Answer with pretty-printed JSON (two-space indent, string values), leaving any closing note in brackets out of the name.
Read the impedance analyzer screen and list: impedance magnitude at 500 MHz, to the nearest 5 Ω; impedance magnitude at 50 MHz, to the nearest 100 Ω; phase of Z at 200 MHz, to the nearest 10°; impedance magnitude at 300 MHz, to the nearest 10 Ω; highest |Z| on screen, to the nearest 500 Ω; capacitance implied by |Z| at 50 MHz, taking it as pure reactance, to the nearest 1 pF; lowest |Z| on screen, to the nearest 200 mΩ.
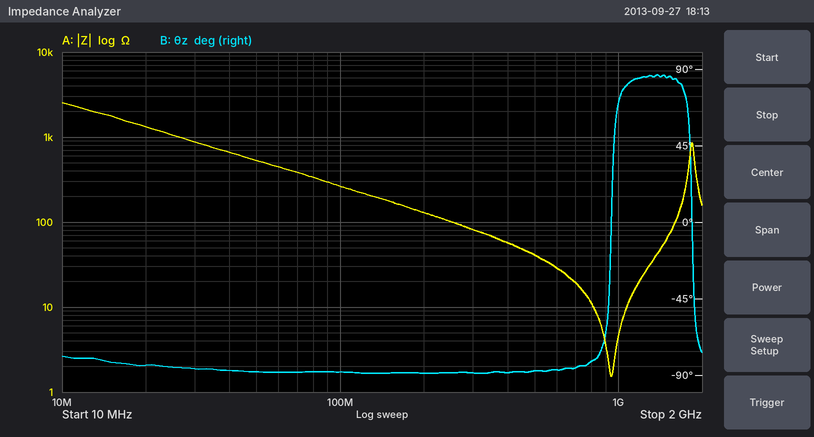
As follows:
{
  "impedance magnitude at 500 MHz, to the nearest 5 Ω": "40 Ω",
  "impedance magnitude at 50 MHz, to the nearest 100 Ω": "500 Ω",
  "phase of Z at 200 MHz, to the nearest 10°": "-90°",
  "impedance magnitude at 300 MHz, to the nearest 10 Ω": "80 Ω",
  "highest |Z| on screen, to the nearest 500 Ω": "2.5 kΩ",
  "capacitance implied by |Z| at 50 MHz, taking it as pure reactance, to the nearest 1 pF": "6 pF",
  "lowest |Z| on screen, to the nearest 200 mΩ": "1.6 Ω"
}
